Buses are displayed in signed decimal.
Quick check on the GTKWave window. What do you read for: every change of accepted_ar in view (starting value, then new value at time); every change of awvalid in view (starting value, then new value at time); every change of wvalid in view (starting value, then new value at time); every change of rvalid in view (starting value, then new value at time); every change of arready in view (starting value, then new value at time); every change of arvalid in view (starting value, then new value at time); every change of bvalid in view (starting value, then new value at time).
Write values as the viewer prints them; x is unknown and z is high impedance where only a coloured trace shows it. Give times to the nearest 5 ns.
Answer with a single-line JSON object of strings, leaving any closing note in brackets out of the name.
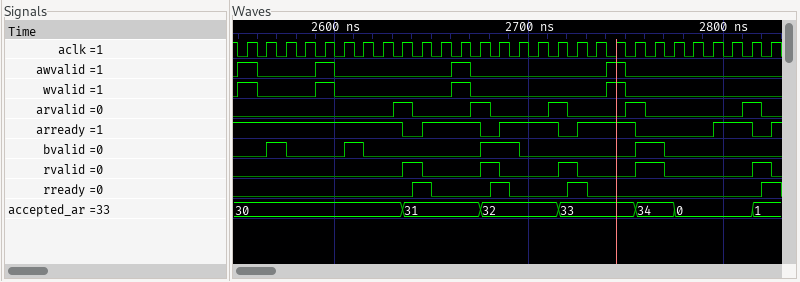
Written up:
{"every change of accepted_ar in view": "30, 31 at 2635 ns, 32 at 2675 ns, 33 at 2715 ns, 34 at 2755 ns, 0 at 2775 ns, 1 at 2815 ns", "every change of awvalid in view": "0, 1 at 2550 ns, 0 at 2560 ns, 1 at 2590 ns, 0 at 2600 ns, 1 at 2660 ns, 0 at 2670 ns, 1 at 2740 ns, 0 at 2750 ns", "every change of wvalid in view": "0, 1 at 2550 ns, 0 at 2560 ns, 1 at 2590 ns, 0 at 2600 ns, 1 at 2660 ns, 0 at 2670 ns, 1 at 2740 ns, 0 at 2750 ns", "every change of rvalid in view": "0, 1 at 2635 ns, 0 at 2645 ns, 1 at 2675 ns, 0 at 2685 ns, 1 at 2715 ns, 0 at 2725 ns, 1 at 2755 ns, 0 at 2770 ns, 1 at 2815 ns, 0 at 2825 ns", "every change of arready in view": "1, 0 at 2635 ns, 1 at 2645 ns, 0 at 2675 ns, 1 at 2685 ns, 0 at 2715 ns, 1 at 2725 ns, 0 at 2755 ns, 1 at 2795 ns, 0 at 2815 ns, 1 at 2825 ns", "every change of arvalid in view": "0, 1 at 2630 ns, 0 at 2640 ns, 1 at 2670 ns, 0 at 2680 ns, 1 at 2710 ns, 0 at 2720 ns, 1 at 2750 ns, 0 at 2760 ns, 1 at 2810 ns, 0 at 2820 ns", "every change of bvalid in view": "0, 1 at 2565 ns, 0 at 2575 ns, 1 at 2605 ns, 0 at 2615 ns, 1 at 2675 ns, 0 at 2695 ns, 1 at 2755 ns, 0 at 2770 ns"}
